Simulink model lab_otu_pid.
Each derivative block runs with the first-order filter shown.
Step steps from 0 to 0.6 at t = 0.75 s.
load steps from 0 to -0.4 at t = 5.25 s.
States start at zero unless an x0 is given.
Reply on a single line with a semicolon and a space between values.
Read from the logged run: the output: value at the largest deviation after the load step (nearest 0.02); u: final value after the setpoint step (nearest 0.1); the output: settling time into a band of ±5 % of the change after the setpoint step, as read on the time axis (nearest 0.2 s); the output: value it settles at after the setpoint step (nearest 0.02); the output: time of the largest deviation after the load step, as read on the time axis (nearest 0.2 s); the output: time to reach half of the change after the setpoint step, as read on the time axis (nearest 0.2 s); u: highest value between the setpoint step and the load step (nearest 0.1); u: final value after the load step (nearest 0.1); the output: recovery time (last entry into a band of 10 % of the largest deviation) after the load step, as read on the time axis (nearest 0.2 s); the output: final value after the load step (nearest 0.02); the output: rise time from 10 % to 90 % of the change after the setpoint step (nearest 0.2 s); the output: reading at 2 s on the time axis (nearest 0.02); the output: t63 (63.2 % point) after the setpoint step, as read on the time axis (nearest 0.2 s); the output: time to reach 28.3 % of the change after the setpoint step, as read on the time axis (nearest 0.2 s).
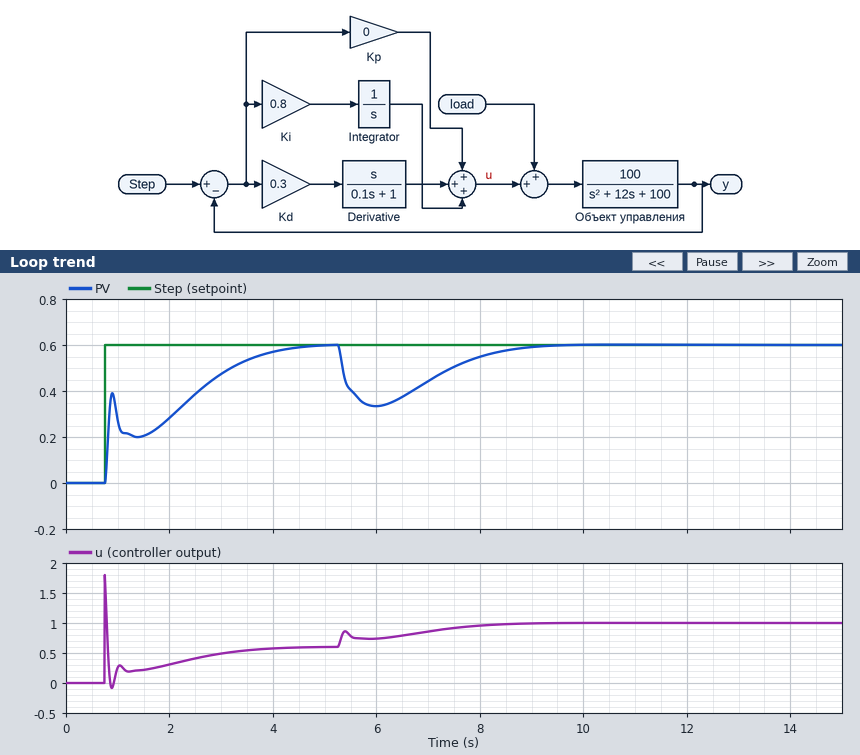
0.34; 0.6; 4.0 s; 0.60; 6.0 s; 0.8 s; 1.8; 1.0; 8.4 s; 0.60; 2.8 s; 0.28; 0.8 s; 0.8 s
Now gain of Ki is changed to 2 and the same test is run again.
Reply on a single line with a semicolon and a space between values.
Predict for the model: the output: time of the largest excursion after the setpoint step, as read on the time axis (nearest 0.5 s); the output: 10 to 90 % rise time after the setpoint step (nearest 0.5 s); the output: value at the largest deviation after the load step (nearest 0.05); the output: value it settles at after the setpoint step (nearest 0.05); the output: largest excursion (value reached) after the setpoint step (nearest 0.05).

3.0 s; 1.5 s; 0.40; 0.60; 0.65
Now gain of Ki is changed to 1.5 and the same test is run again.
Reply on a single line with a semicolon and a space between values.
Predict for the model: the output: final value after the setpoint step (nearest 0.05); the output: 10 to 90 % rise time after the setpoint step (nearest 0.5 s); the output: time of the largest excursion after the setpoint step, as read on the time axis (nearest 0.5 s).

0.60; 1.5 s; 3.5 s
